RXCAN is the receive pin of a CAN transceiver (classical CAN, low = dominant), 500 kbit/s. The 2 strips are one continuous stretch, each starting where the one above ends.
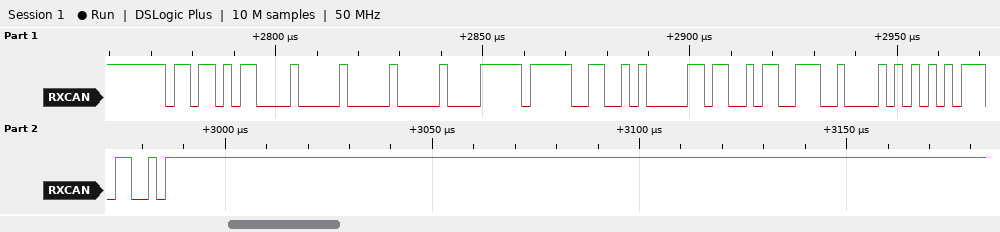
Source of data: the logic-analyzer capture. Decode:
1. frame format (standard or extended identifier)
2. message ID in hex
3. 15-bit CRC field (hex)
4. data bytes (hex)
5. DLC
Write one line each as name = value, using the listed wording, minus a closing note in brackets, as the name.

frame format = standard
message ID in hex = 0x6D6
15-bit CRC field = 0x2AEC
data bytes = 00 00 FF D9 41 65 9C 85
DLC = 8
